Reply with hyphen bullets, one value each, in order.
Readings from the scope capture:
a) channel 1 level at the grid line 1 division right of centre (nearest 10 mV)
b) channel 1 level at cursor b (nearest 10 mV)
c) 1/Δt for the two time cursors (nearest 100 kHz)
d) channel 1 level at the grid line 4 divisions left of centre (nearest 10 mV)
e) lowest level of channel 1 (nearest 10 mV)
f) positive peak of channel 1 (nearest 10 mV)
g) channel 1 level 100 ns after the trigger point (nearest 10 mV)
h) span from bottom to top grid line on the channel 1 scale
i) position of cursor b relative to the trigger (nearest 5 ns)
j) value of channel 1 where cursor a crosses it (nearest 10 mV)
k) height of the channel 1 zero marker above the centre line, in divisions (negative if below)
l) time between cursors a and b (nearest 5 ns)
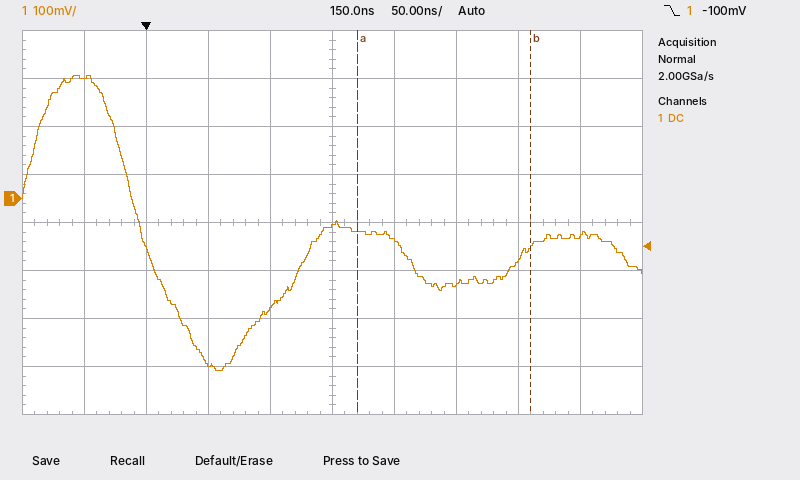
- -90 mV
- -100 mV
- 7.1 MHz
- 250 mV
- -360 mV
- 260 mV
- -230 mV
- 800 mV
- +310 ns
- -70 mV
- +0.5 div
- 140 ns
